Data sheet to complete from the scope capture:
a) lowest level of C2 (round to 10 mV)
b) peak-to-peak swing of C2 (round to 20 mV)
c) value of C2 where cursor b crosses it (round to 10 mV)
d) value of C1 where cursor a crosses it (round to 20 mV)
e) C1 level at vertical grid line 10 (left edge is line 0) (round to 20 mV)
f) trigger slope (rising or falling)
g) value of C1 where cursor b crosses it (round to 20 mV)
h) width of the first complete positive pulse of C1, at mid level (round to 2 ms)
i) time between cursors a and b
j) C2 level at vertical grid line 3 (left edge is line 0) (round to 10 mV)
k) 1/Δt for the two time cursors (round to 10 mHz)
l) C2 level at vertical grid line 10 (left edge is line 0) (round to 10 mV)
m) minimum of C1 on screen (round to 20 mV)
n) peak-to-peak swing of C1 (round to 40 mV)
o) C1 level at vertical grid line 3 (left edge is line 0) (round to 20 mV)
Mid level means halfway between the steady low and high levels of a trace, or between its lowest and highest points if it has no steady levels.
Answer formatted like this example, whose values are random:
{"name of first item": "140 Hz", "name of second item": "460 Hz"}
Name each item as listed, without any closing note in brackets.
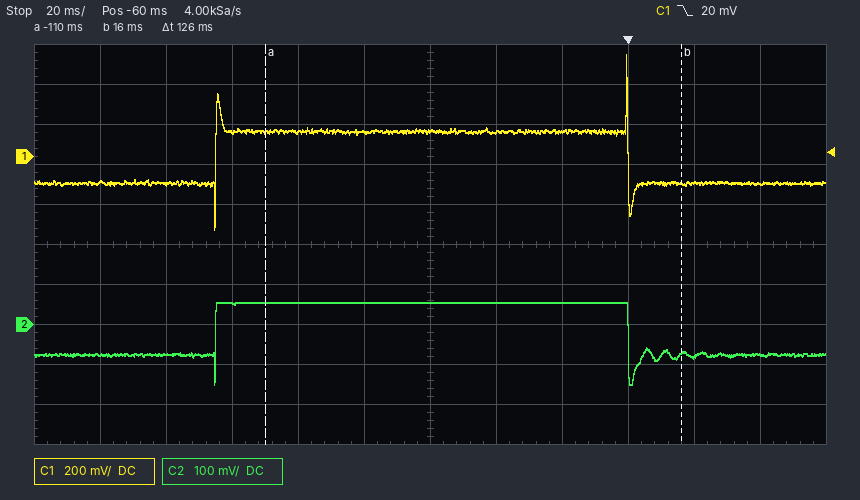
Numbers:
{"lowest level of C2": "-150 mV", "peak-to-peak swing of C2": "200 mV", "value of C2 where cursor b crosses it": "-70 mV", "value of C1 where cursor a crosses it": "120 mV", "C1 level at vertical grid line 10 (left edge is line 0)": "-140 mV", "trigger slope": "falling", "value of C1 where cursor b crosses it": "-140 mV", "width of the first complete positive pulse of C1, at mid level": "124 ms", "time between cursors a and b": "126 ms", "C2 level at vertical grid line 3 (left edge is line 0)": "50 mV", "1/Δt for the two time cursors": "7.94 Hz", "C2 level at vertical grid line 10 (left edge is line 0)": "-80 mV", "minimum of C1 on screen": "-360 mV", "peak-to-peak swing of C1": "880 mV", "C1 level at vertical grid line 3 (left edge is line 0)": "120 mV"}
